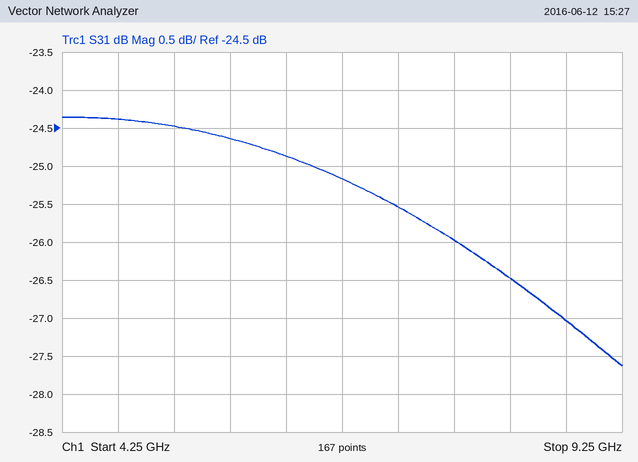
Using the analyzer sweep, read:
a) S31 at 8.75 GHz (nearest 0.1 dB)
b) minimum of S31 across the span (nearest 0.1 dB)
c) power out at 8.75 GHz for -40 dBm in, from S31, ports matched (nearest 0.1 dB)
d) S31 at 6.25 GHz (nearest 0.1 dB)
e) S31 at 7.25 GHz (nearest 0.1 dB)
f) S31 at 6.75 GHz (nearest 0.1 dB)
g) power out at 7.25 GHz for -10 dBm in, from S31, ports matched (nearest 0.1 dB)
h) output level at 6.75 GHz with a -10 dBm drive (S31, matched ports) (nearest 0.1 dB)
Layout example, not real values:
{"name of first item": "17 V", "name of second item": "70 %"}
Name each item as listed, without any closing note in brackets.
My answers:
{"S31 at 8.75 GHz": "-27.0 dB", "minimum of S31 across the span": "-27.6 dB", "power out at 8.75 GHz for -40 dBm in, from S31, ports matched": "-67.0 dBm", "S31 at 6.25 GHz": "-24.9 dB", "S31 at 7.25 GHz": "-25.5 dB", "S31 at 6.75 GHz": "-25.2 dB", "power out at 7.25 GHz for -10 dBm in, from S31, ports matched": "-35.5 dBm", "output level at 6.75 GHz with a -10 dBm drive (S31, matched ports)": "-35.2 dBm"}
